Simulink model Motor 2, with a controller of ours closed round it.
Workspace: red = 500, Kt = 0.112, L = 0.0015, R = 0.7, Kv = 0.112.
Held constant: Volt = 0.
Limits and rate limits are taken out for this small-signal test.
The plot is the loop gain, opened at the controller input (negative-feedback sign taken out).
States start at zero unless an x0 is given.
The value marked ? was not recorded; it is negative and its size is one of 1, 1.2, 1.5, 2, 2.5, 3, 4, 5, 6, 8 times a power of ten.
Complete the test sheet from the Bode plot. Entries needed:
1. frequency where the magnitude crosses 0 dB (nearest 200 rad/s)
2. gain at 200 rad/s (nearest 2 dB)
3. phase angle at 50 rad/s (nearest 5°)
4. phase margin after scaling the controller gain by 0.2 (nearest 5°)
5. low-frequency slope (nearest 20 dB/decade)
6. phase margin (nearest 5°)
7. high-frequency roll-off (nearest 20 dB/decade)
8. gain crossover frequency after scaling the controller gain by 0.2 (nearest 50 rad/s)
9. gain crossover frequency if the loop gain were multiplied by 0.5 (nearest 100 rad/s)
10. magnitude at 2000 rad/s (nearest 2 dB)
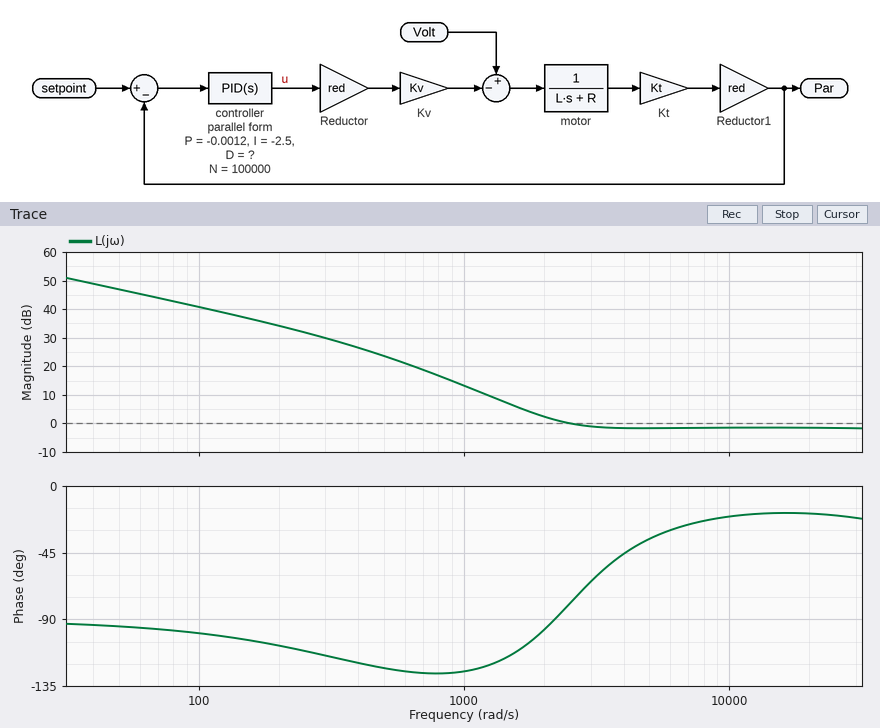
2600 rad/s
34 dB
-95°
55°
-20 dB/decade
100°
0 dB/decade
950 rad/s
1600 rad/s
2 dB
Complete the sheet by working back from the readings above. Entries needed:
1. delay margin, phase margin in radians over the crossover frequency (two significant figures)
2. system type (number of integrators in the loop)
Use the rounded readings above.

0.00067 s
1
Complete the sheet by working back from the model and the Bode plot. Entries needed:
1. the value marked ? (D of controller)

-4e-07
